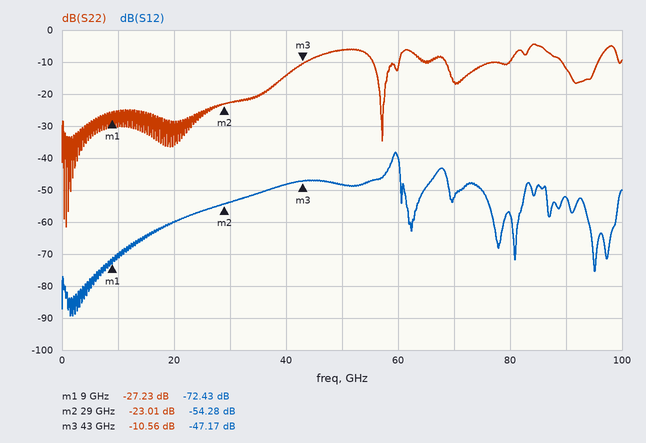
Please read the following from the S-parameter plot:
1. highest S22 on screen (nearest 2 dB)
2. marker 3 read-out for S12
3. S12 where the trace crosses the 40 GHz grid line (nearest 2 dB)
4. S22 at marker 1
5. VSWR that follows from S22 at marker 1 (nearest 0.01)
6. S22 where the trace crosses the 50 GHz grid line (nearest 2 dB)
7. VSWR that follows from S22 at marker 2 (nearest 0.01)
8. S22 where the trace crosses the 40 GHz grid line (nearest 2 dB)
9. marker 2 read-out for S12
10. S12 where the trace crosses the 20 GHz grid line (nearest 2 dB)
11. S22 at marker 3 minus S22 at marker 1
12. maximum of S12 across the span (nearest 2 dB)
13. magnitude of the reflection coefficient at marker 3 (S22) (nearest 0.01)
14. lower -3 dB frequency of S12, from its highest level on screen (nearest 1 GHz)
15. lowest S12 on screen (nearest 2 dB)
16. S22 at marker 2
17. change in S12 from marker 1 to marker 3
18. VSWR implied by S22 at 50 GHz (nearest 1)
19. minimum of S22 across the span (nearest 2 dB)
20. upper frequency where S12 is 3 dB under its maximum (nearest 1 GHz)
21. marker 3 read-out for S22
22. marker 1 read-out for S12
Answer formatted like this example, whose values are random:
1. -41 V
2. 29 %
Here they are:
1. -4 dB
2. -47.17 dB
3. -48 dB
4. -27.23 dB
5. 1.09
6. -6 dB
7. 1.15
8. -14 dB
9. -54.28 dB
10. -60 dB
11. 16.67 dB
12. -38 dB
13. 0.30
14. 59 GHz
15. -90 dB
16. -23.01 dB
17. 25.26 dB
18. 3
19. -62 dB
20. 60 GHz
21. -10.56 dB
22. -72.43 dB
